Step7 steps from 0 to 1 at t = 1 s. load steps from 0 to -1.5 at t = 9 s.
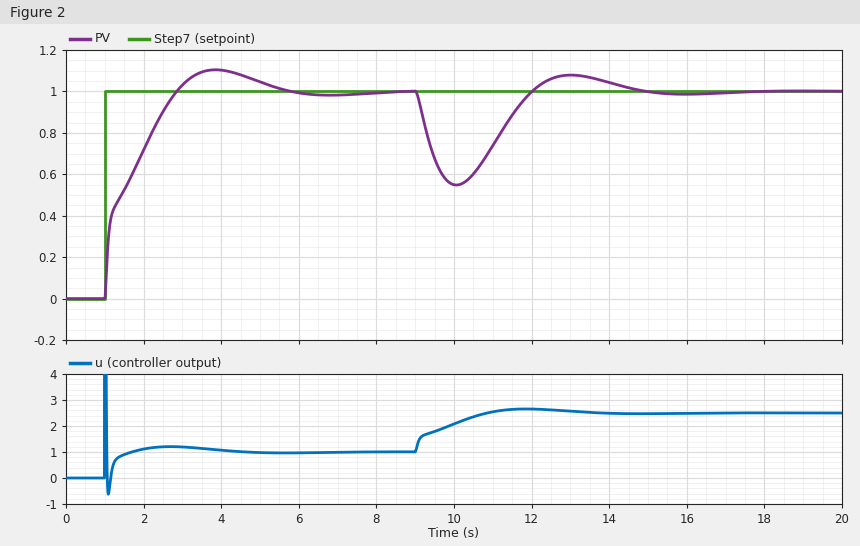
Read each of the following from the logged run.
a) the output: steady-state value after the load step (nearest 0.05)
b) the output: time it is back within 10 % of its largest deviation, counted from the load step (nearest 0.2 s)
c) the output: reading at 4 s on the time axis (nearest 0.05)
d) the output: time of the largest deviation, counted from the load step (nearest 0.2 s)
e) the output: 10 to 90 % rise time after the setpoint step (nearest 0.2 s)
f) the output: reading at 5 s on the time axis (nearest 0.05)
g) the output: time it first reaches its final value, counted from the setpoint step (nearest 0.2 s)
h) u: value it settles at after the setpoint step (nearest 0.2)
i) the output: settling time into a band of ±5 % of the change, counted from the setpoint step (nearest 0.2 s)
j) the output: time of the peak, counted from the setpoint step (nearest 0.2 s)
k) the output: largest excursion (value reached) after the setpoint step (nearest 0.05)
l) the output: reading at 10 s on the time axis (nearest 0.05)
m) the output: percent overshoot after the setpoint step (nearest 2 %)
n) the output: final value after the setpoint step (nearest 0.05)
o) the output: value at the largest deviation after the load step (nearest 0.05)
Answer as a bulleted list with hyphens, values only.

- 1.00
- 5.0 s
- 1.10
- 1.0 s
- 1.4 s
- 1.05
- 1.8 s
- 1.0
- 4.0 s
- 2.8 s
- 1.10
- 0.55
- 10 %
- 1.00
- 0.55
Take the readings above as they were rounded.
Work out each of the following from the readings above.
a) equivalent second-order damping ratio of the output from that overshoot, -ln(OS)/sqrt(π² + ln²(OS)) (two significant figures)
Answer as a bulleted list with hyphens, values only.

- 0.59
